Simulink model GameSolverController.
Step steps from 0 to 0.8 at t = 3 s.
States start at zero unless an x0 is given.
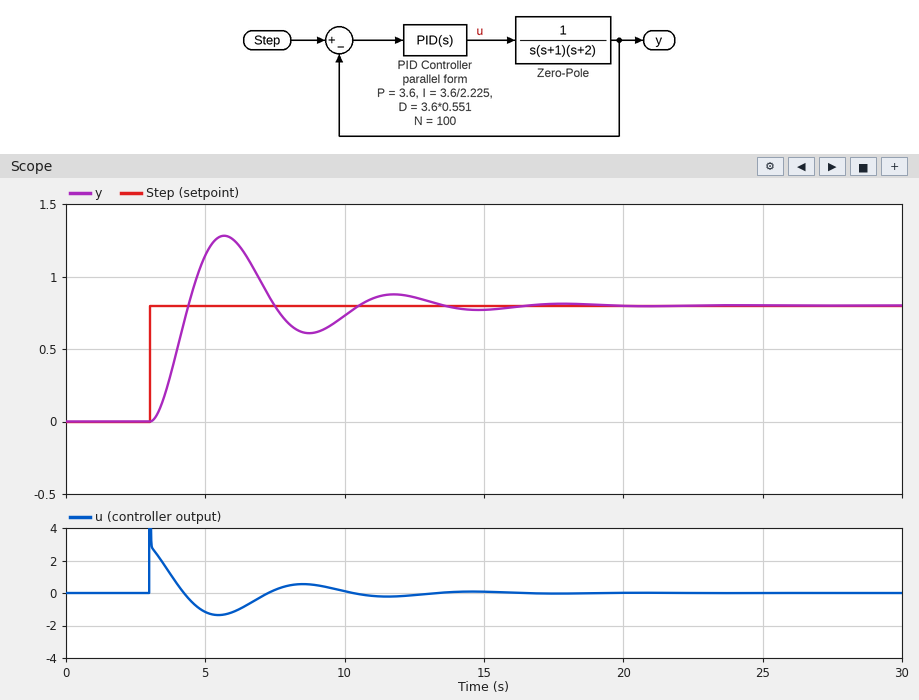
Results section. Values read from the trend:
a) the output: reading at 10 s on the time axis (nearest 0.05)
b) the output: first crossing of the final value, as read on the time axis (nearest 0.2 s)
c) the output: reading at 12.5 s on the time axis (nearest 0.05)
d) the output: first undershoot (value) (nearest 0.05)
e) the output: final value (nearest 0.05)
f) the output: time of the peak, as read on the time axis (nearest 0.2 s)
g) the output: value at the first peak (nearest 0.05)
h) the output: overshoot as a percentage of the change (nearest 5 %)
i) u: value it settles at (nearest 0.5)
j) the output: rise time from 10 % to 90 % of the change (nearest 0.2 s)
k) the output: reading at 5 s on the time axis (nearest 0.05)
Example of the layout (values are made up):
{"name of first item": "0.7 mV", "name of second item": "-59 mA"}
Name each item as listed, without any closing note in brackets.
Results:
{"the output: reading at 10 s on the time axis": "0.75", "the output: first crossing of the final value, as read on the time axis": "4.4 s", "the output: reading at 12.5 s on the time axis": "0.85", "the output: first undershoot (value)": "0.60", "the output: final value": "0.80", "the output: time of the peak, as read on the time axis": "5.6 s", "the output: value at the first peak": "1.30", "the output: overshoot as a percentage of the change": "60 %", "u: value it settles at": "0.0", "the output: rise time from 10 % to 90 % of the change": "1.0 s", "the output: reading at 5 s on the time axis": "1.15"}
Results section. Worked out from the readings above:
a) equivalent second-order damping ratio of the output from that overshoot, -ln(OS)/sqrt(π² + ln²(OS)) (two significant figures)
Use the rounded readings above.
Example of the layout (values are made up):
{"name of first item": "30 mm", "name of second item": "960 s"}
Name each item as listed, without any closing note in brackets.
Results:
{"equivalent second-order damping ratio of the output from that overshoot, -ln(OS)/sqrt(π² + ln²(OS))": "0.16"}
